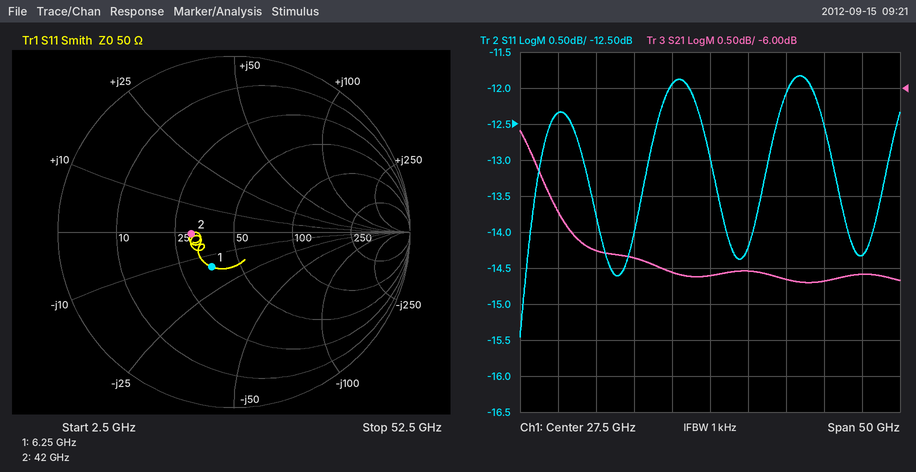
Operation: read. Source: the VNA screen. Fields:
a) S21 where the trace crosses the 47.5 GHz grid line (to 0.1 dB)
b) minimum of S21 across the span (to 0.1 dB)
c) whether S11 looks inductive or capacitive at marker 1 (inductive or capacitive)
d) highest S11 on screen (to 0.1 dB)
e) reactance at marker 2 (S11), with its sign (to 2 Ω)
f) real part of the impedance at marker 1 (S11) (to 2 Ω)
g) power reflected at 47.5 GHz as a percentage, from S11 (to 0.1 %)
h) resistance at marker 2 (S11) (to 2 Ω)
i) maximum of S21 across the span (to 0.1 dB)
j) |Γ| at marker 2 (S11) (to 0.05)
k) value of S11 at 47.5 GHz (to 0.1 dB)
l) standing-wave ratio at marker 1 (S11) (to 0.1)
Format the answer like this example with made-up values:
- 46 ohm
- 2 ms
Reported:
- -8.6 dB
- -8.7 dB
- capacitive
- -11.8 dB
- 0 Ω
- 36 Ω
- 3.7 %
- 30 Ω
- -6.6 dB
- 0.25
- -14.3 dB
- 1.6
